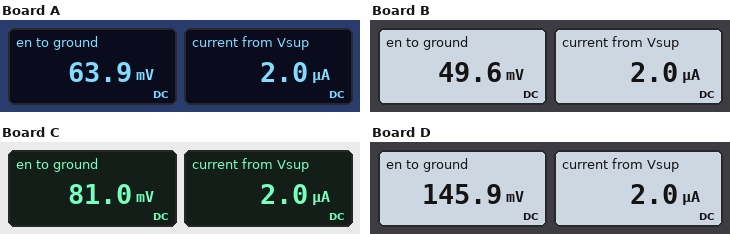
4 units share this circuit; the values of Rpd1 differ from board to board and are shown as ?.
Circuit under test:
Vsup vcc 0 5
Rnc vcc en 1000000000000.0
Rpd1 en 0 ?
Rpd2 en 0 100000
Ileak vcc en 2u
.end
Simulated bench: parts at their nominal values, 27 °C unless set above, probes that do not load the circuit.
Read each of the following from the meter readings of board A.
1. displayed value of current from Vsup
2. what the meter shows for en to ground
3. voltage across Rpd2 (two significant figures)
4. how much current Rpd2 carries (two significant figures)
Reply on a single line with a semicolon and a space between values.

2.0 µA; 63.9 mV; 64 mV; 640 nA
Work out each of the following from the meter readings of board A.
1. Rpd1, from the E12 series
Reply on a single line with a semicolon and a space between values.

47 kΩ
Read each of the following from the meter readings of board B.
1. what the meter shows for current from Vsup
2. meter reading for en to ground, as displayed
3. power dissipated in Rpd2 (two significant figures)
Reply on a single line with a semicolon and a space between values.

2.0 µA; 49.6 mV; 25 nW
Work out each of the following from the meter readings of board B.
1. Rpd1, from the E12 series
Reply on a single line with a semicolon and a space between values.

33 kΩ
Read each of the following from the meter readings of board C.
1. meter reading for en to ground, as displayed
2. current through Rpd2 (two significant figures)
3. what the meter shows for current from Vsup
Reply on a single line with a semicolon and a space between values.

81.0 mV; 810 nA; 2.0 µA
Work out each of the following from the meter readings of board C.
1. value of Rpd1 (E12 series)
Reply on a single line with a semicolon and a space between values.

68 kΩ
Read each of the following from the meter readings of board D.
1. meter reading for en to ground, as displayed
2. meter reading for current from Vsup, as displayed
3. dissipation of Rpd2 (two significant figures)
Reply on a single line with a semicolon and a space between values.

145.9 mV; 2.0 µA; 210 nW
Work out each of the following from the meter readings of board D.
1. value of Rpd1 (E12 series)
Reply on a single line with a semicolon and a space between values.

270 kΩ
